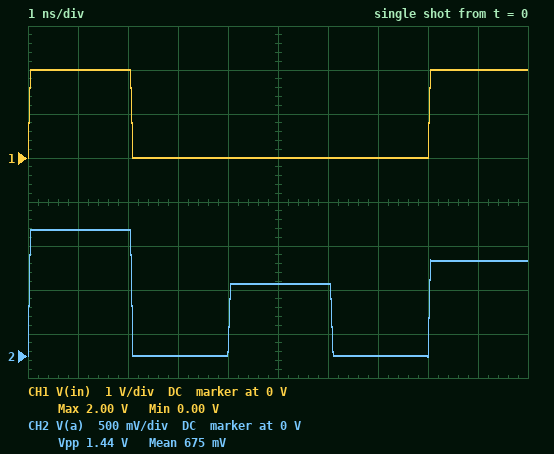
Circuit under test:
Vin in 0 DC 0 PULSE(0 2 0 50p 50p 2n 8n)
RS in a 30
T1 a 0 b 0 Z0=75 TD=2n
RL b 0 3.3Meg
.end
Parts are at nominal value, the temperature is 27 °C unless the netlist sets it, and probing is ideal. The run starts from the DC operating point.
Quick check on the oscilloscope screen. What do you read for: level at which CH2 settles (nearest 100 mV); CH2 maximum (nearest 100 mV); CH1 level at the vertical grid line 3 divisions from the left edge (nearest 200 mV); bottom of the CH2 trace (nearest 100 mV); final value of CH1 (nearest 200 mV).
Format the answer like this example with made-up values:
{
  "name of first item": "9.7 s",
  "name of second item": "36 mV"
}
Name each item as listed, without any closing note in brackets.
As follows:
{
  "level at which CH2 settles": "1.1 V",
  "CH2 maximum": "1.4 V",
  "CH1 level at the vertical grid line 3 divisions from the left edge": "0 V",
  "bottom of the CH2 trace": "0 V",
  "final value of CH1": "2.0 V"
}
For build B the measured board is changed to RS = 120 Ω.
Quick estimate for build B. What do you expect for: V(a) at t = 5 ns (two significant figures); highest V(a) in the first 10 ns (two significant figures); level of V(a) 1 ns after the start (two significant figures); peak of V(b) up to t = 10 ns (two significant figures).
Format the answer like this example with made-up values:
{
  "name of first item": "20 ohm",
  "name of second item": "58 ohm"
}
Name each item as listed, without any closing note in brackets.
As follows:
{
  "V(a) at t = 5 ns": "950 mV",
  "highest V(a) in the first 10 ns": "990 mV",
  "level of V(a) 1 ns after the start": "770 mV",
  "peak of V(b) up to t = 10 ns": "1.5 V"
}
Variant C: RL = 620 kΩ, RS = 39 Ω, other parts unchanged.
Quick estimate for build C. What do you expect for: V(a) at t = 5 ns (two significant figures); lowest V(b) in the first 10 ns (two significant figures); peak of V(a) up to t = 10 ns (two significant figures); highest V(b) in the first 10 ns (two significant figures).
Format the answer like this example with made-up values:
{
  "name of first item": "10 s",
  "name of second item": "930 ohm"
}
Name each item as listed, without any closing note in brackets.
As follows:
{
  "V(a) at t = 5 ns": "900 mV",
  "lowest V(b) in the first 10 ns": "-830 mV",
  "peak of V(a) up to t = 10 ns": "1.3 V",
  "highest V(b) in the first 10 ns": "2.6 V"
}
